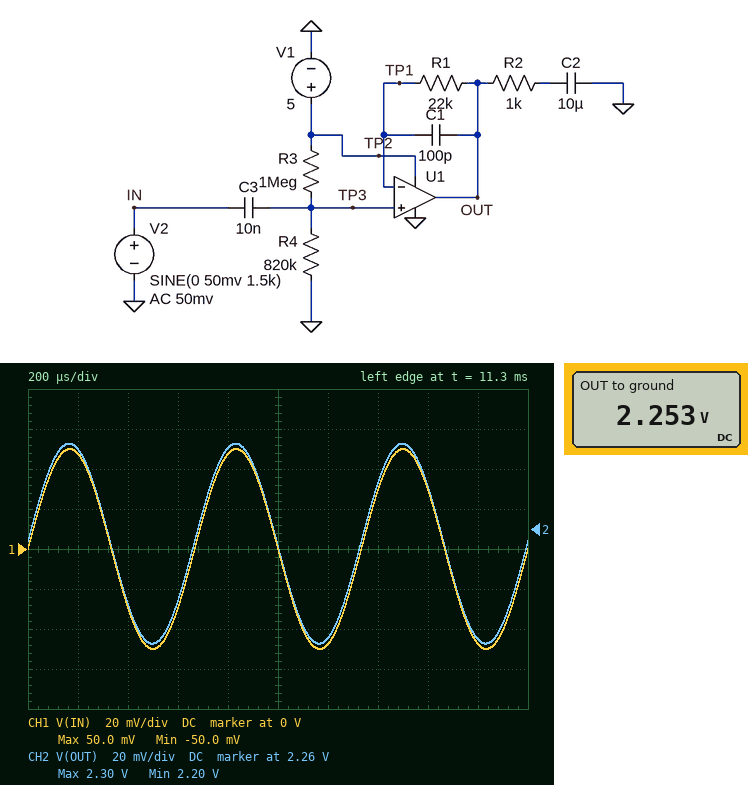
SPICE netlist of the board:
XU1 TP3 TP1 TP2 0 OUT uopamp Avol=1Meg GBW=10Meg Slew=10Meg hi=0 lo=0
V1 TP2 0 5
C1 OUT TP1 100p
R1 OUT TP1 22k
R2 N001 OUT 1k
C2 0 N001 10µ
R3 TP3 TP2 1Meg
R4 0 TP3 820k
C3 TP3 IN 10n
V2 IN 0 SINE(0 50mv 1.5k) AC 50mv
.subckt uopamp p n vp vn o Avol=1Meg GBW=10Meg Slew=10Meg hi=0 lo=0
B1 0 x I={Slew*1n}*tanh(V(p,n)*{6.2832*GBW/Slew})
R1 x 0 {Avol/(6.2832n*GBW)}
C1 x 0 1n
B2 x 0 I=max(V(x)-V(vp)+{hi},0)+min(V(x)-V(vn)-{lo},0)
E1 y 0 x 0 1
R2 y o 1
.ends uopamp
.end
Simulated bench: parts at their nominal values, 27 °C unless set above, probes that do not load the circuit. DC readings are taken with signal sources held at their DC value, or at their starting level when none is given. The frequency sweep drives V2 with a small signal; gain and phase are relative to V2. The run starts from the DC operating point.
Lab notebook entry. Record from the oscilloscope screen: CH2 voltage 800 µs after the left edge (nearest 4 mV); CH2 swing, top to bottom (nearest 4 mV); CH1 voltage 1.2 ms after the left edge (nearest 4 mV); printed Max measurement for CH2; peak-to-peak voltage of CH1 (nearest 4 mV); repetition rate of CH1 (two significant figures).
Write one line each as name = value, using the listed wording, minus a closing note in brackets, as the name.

CH2 voltage 800 µs after the left edge = 2.300 V
CH2 swing, top to bottom = 100 mV
CH1 voltage 1.2 ms after the left edge = -48 mV
printed Max measurement for CH2 = 2.30 V
peak-to-peak voltage of CH1 = 100 mV
repetition rate of CH1 = 1.5 kHz
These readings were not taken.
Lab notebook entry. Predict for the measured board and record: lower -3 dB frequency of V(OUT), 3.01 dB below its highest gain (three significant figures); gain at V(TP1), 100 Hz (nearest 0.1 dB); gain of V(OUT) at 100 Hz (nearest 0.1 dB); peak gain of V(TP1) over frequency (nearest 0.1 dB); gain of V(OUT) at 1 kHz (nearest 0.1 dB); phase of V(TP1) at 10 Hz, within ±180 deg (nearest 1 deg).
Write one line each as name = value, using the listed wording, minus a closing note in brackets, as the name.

lower -3 dB frequency of V(OUT), 3.01 dB below its highest gain = 35.3 Hz
gain at V(TP1), 100 Hz = -0.5 dB
gain of V(OUT) at 100 Hz = -0.5 dB
peak gain of V(TP1) over frequency = 0 dB
gain of V(OUT) at 1 kHz = 0 dB
phase of V(TP1) at 10 Hz, within ±180 deg = 74 deg
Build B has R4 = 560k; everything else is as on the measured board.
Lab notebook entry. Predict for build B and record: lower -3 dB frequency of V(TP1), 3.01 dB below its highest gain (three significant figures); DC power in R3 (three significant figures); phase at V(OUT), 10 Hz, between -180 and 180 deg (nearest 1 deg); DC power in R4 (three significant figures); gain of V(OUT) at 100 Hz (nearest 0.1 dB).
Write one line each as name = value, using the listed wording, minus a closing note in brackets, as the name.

lower -3 dB frequency of V(TP1), 3.01 dB below its highest gain = 44.3 Hz
DC power in R3 = 10.3 µW
phase at V(OUT), 10 Hz, between -180 and 180 deg = 77 deg
DC power in R4 = 5.75 µW
gain of V(OUT) at 100 Hz = -0.8 dB
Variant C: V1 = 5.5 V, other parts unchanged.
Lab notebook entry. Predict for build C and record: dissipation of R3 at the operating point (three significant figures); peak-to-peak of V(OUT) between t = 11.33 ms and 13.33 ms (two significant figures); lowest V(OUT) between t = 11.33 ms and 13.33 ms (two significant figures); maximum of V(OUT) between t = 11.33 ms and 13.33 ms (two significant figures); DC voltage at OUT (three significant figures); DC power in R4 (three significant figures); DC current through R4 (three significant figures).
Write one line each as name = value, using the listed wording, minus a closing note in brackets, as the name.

dissipation of R3 at the operating point = 9.13 µW
peak-to-peak of V(OUT) between t = 11.33 ms and 13.33 ms = 100 mV
lowest V(OUT) between t = 11.33 ms and 13.33 ms = 2.4 V
maximum of V(OUT) between t = 11.33 ms and 13.33 ms = 2.5 V
DC voltage at OUT = 2.48 V
DC power in R4 = 7.49 µW
DC current through R4 = 3.02 µA
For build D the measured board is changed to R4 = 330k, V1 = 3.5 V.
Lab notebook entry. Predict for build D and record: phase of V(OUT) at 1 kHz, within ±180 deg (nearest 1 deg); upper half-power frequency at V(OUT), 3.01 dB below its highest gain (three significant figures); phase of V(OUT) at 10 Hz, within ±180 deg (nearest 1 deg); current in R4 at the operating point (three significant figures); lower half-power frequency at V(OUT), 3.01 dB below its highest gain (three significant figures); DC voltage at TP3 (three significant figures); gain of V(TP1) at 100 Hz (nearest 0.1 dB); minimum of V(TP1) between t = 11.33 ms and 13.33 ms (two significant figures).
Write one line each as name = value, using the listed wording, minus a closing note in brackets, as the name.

phase of V(OUT) at 1 kHz, within ±180 deg = 4 deg
upper half-power frequency at V(OUT), 3.01 dB below its highest gain = 9.99 MHz
phase of V(OUT) at 10 Hz, within ±180 deg = 81 deg
current in R4 at the operating point = 2.63 µA
lower half-power frequency at V(OUT), 3.01 dB below its highest gain = 64.1 Hz
DC voltage at TP3 = 868 mV
gain of V(TP1) at 100 Hz = -1.5 dB
minimum of V(TP1) between t = 11.33 ms and 13.33 ms = 820 mV
